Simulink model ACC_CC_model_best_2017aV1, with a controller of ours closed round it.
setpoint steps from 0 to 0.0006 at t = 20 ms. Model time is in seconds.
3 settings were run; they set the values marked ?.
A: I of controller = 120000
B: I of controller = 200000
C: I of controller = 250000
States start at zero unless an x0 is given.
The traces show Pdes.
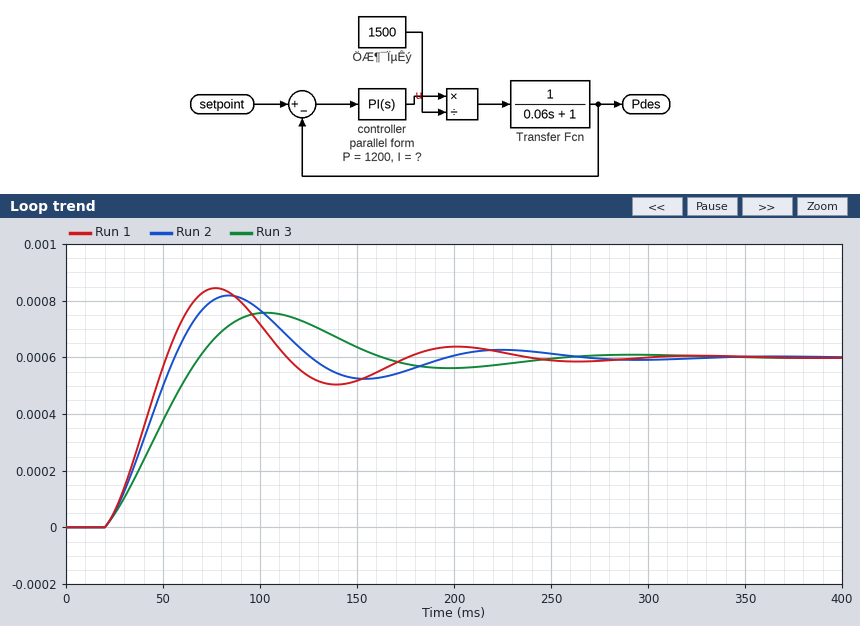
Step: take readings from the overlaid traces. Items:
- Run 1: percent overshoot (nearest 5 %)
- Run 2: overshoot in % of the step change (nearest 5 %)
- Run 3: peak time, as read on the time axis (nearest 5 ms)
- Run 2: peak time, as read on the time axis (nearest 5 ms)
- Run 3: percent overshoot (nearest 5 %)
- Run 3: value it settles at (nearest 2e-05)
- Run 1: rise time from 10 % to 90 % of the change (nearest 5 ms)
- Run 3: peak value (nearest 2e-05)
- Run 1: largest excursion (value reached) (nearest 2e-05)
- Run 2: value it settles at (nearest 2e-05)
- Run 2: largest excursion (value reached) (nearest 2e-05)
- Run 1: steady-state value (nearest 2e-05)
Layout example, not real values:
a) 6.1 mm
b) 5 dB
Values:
a) 40 %
b) 35 %
c) 105 ms
d) 85 ms
e) 25 %
f) 0.00060
g) 25 ms
h) 0.00076
i) 0.00084
j) 0.00060
k) 0.00082
l) 0.00060
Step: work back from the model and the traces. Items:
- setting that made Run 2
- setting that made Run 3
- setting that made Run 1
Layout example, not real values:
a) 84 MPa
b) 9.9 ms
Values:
a) B
b) A
c) C
